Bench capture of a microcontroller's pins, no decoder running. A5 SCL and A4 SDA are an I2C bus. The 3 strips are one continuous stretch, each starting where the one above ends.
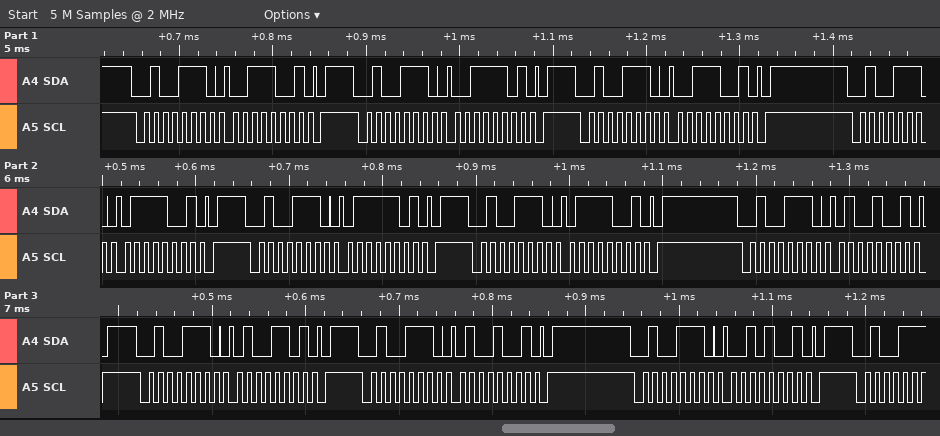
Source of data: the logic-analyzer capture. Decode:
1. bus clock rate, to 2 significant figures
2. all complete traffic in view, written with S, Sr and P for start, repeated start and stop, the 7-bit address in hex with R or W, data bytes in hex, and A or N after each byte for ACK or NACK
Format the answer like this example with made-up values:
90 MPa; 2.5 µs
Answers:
100 kHz; S 27W A 39 A P S 27W A 3D A P S 27W A 39 A P S 27W A 79 A P S 27W A 7D A P S 27W A 79 A P S 27W A 49 A P S 27W A 4D A P S 27W A 49 A P S 27W A 29 A P
